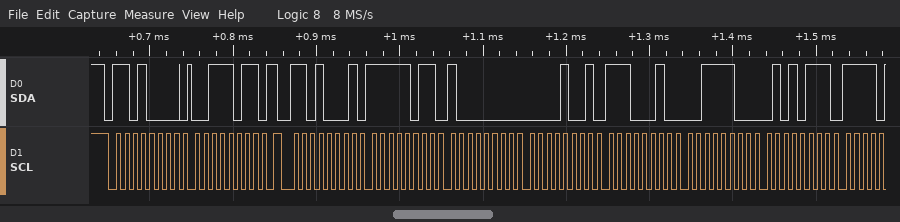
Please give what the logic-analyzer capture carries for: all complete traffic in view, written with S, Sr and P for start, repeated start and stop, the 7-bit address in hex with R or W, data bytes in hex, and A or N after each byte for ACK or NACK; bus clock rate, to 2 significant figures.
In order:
S 68W A 3B A Sr 68R A FB A 80 A 09 A E2 A 3C A 57 A
100 kHz
